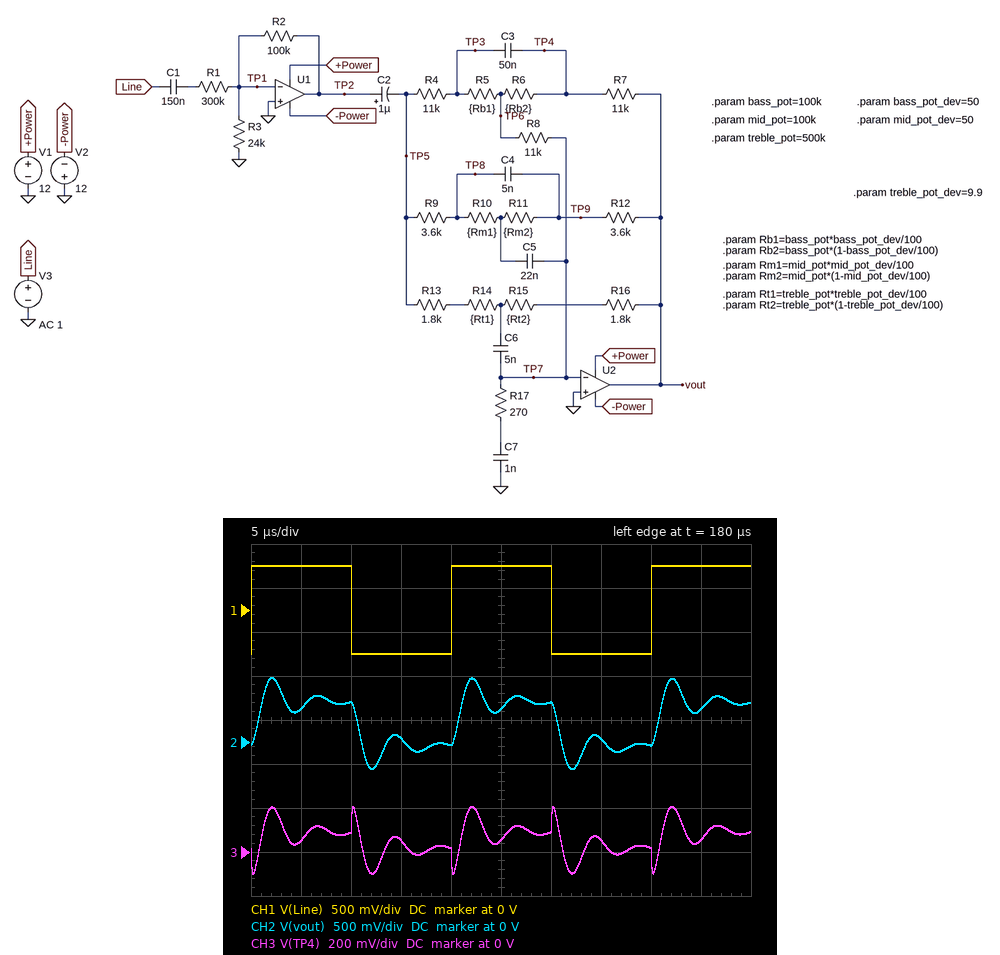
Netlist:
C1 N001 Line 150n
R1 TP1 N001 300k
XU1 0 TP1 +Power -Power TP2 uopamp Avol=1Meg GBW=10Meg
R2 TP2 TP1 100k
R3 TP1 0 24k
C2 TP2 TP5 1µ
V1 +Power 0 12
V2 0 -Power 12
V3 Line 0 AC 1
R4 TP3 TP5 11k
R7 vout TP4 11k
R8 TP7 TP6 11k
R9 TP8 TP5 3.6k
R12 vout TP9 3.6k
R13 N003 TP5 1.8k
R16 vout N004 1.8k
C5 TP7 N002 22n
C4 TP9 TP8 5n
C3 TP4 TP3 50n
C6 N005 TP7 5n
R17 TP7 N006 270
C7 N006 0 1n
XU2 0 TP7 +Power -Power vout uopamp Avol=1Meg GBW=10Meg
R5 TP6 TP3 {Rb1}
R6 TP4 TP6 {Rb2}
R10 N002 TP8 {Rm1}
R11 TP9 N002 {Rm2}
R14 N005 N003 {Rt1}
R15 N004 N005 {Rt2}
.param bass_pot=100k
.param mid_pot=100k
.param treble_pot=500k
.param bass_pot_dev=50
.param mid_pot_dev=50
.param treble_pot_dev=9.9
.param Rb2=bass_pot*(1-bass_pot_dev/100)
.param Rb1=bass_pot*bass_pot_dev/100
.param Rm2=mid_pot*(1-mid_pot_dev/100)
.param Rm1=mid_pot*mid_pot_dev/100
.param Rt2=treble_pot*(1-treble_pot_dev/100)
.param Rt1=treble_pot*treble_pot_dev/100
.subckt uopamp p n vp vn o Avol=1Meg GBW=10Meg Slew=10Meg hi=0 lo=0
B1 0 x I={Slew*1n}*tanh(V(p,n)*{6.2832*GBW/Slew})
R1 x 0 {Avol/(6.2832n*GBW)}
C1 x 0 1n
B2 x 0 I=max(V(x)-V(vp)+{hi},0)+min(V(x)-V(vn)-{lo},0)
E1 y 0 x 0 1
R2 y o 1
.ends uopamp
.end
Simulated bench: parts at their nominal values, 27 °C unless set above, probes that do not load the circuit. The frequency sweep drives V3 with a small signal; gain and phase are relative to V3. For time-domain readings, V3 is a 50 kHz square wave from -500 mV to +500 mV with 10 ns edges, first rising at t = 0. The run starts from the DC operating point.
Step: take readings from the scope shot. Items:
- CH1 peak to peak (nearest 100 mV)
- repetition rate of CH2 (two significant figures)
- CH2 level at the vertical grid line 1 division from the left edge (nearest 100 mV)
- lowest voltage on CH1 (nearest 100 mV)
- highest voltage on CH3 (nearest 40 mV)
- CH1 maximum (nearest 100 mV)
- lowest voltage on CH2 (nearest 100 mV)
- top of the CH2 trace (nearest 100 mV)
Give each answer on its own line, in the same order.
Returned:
1.0 V
50 kHz
400 mV
-500 mV
200 mV
500 mV
-300 mV
700 mV
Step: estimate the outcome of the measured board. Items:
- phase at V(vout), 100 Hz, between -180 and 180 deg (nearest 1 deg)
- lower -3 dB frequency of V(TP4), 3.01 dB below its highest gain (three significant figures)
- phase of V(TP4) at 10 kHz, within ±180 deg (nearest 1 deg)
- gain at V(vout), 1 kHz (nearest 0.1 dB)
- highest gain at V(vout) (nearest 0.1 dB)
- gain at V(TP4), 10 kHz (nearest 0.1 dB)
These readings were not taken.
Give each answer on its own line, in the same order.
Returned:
14 deg
185 kHz
-2 deg
-6.6 dB
1.9 dB
-22.4 dB
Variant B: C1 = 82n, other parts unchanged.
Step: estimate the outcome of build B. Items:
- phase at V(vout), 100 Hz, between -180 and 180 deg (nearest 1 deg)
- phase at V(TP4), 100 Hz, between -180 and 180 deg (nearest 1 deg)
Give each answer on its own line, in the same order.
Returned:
16 deg
-12 deg
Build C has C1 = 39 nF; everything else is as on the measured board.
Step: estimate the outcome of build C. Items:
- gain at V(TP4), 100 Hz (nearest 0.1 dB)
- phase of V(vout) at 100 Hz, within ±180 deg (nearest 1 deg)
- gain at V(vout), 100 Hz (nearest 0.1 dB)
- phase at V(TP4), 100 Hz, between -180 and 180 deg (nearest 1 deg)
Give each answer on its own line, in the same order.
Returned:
-12.7 dB
20 deg
-9.5 dB
-8 deg
